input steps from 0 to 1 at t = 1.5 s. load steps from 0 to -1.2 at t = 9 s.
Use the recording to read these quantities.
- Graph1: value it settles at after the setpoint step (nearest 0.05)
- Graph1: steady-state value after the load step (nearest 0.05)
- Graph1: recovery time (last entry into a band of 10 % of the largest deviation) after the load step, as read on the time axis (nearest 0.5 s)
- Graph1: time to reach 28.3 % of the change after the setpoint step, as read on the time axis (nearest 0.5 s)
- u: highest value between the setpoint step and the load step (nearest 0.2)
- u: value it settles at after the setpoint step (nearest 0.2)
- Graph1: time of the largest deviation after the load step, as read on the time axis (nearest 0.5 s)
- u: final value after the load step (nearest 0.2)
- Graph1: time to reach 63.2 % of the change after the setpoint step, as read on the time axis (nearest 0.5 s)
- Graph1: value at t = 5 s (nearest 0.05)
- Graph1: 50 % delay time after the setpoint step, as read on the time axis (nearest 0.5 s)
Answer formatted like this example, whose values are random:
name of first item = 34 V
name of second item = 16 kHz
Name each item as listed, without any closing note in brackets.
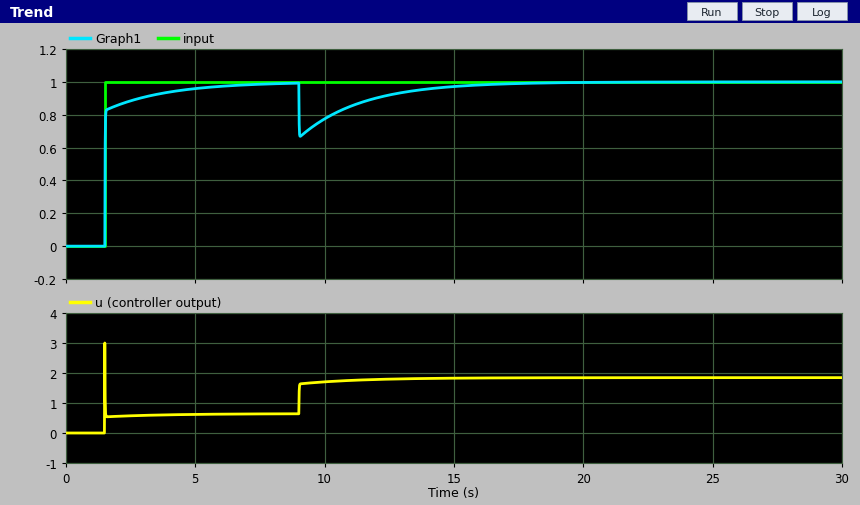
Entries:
Graph1: value it settles at after the setpoint step = 1.00
Graph1: steady-state value after the load step = 1.00
Graph1: recovery time (last entry into a band of 10 % of the largest deviation) after the load step, as read on the time axis = 14.5 s
Graph1: time to reach 28.3 % of the change after the setpoint step, as read on the time axis = 1.5 s
u: highest value between the setpoint step and the load step = 3.0
u: value it settles at after the setpoint step = 0.6
Graph1: time of the largest deviation after the load step, as read on the time axis = 9.0 s
u: final value after the load step = 1.8
Graph1: time to reach 63.2 % of the change after the setpoint step, as read on the time axis = 1.5 s
Graph1: value at t = 5 s = 0.95
Graph1: 50 % delay time after the setpoint step, as read on the time axis = 1.5 s
